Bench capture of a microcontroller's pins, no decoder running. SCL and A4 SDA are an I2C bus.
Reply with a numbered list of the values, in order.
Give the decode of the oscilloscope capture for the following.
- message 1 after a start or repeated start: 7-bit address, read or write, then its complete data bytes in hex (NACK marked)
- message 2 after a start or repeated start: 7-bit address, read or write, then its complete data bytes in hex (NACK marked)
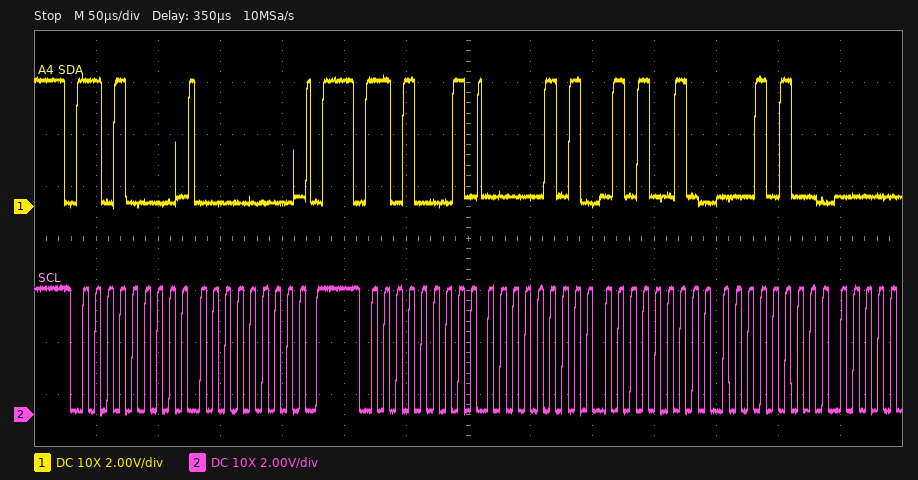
1. 0x68 write: 00
2. 0x68 read: 05 52 14
